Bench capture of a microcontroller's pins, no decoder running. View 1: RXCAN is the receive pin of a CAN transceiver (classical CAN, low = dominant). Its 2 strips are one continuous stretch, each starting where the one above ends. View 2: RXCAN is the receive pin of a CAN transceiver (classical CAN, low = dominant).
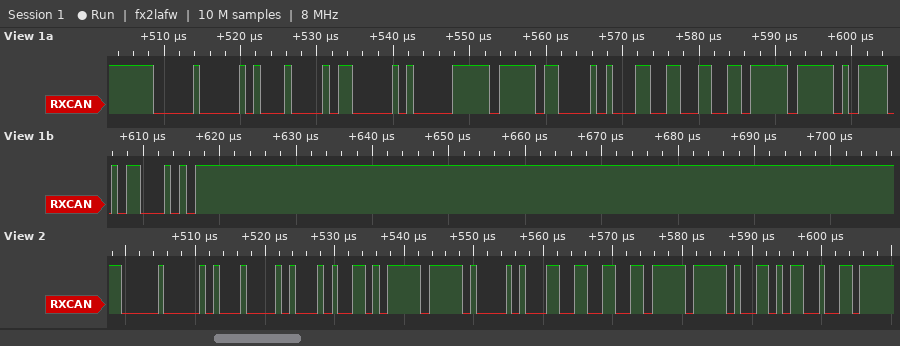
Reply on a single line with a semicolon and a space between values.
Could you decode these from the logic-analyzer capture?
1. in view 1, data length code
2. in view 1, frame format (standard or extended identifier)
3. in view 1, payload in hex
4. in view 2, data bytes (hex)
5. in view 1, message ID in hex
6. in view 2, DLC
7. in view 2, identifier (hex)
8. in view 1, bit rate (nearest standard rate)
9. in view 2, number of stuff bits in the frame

8; standard; 58 10 7F F0 A3 33 37 FF; 51 4D 7F F0 A3 33 37 FF; 0x001; 8; 0x001; 1000 kbit/s; 6
